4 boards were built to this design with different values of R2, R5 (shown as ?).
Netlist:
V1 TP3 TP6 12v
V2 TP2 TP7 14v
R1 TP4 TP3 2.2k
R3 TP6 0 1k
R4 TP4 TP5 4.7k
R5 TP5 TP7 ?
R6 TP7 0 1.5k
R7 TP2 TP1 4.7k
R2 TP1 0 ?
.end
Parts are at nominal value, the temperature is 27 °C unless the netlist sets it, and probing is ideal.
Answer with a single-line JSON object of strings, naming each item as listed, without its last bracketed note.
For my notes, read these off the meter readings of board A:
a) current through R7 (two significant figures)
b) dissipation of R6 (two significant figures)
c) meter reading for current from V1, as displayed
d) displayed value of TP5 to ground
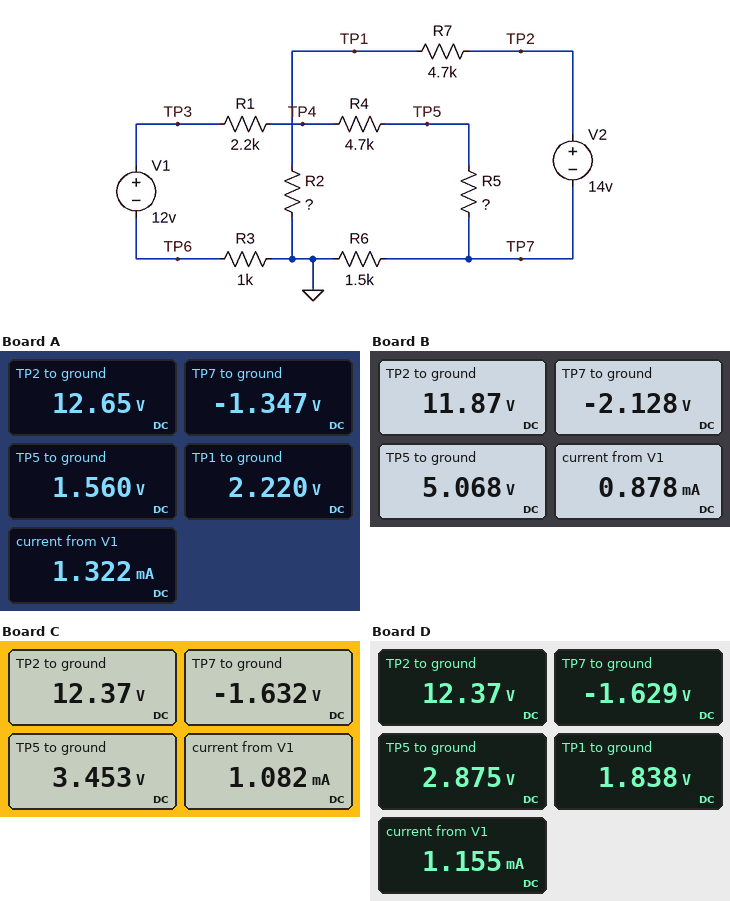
{"current through R7": "2.2 mA", "dissipation of R6": "1.2 mW", "meter reading for current from V1, as displayed": "1.322 mA", "displayed value of TP5 to ground": "1.560 V"}
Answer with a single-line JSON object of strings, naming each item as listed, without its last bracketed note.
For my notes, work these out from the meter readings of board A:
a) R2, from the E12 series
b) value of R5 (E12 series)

{"R2, from the E12 series": "1 kΩ", "value of R5": "2.2 kΩ"}
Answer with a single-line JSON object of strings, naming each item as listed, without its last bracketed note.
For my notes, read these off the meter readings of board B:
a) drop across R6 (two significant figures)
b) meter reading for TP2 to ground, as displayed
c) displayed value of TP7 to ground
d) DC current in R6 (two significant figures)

{"drop across R6": "2.1 V", "meter reading for TP2 to ground, as displayed": "11.87 V", "displayed value of TP7 to ground": "-2.128 V", "DC current in R6": "1.4 mA"}
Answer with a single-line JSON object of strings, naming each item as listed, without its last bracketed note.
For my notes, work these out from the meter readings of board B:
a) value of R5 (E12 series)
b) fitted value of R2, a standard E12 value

{"value of R5": "8.2 kΩ", "fitted value of R2, a standard E12 value": "470 Ω"}
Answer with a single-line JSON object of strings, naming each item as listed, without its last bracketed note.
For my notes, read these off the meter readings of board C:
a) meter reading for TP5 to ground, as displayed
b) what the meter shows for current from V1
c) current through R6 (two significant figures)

{"meter reading for TP5 to ground, as displayed": "3.453 V", "what the meter shows for current from V1": "1.082 mA", "current through R6": "1.1 mA"}
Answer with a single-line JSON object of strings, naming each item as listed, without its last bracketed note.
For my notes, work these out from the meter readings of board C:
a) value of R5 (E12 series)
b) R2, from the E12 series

{"value of R5": "4.7 kΩ", "R2, from the E12 series": "1 kΩ"}
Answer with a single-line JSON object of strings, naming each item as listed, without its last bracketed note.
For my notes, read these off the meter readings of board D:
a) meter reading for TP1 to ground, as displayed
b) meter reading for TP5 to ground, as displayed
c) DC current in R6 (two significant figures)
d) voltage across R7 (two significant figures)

{"meter reading for TP1 to ground, as displayed": "1.838 V", "meter reading for TP5 to ground, as displayed": "2.875 V", "DC current in R6": "1.1 mA", "voltage across R7": "11 V"}
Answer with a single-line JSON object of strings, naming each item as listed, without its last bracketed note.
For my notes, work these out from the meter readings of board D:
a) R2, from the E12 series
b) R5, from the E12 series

{"R2, from the E12 series": "820 Ω", "R5, from the E12 series": "3.9 kΩ"}
